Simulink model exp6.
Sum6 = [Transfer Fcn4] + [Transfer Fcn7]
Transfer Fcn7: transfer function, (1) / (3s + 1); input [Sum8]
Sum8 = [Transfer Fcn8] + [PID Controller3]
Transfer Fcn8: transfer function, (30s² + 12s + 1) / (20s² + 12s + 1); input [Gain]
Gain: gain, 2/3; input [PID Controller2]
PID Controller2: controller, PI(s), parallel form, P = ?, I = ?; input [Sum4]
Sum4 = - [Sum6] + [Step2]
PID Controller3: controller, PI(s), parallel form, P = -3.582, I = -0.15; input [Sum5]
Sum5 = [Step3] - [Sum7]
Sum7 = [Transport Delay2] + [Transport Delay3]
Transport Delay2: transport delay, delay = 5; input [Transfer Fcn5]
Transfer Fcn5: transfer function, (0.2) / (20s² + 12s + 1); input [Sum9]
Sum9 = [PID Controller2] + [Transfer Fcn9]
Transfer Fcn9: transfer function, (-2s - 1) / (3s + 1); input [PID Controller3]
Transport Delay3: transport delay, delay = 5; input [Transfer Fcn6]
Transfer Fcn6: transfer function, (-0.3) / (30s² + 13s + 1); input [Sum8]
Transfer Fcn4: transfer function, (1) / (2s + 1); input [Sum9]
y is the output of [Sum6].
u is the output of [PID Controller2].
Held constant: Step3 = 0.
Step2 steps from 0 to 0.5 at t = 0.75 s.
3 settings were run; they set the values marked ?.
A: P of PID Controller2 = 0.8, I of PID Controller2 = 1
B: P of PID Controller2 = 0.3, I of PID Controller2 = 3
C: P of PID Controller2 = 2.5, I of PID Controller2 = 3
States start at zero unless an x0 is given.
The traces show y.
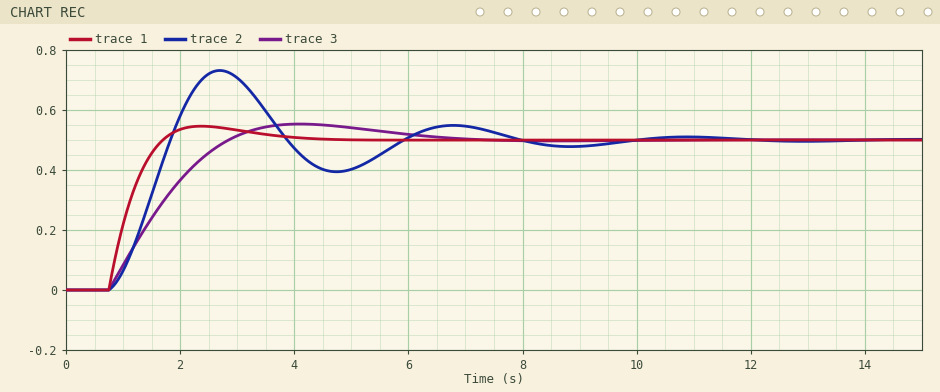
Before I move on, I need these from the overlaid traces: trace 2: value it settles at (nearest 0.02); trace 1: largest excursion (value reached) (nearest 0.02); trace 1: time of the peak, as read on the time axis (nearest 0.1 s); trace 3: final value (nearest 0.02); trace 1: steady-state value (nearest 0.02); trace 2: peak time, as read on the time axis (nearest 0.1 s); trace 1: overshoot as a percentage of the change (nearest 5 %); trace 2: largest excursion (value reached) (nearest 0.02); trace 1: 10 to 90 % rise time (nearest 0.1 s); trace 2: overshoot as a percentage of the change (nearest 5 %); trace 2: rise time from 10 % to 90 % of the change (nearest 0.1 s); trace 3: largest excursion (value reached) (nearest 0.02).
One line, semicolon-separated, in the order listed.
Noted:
0.50; 0.54; 2.4 s; 0.50; 0.50; 2.7 s; 10 %; 0.74; 0.7 s; 45 %; 0.8 s; 0.56
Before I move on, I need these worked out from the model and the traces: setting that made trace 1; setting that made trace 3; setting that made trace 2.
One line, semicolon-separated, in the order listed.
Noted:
C; A; B
